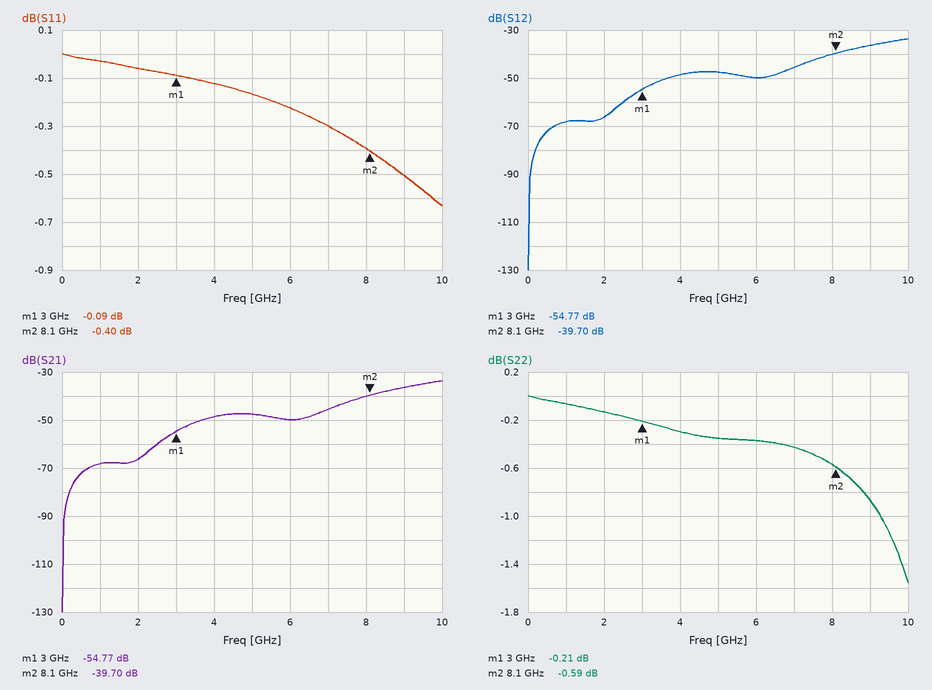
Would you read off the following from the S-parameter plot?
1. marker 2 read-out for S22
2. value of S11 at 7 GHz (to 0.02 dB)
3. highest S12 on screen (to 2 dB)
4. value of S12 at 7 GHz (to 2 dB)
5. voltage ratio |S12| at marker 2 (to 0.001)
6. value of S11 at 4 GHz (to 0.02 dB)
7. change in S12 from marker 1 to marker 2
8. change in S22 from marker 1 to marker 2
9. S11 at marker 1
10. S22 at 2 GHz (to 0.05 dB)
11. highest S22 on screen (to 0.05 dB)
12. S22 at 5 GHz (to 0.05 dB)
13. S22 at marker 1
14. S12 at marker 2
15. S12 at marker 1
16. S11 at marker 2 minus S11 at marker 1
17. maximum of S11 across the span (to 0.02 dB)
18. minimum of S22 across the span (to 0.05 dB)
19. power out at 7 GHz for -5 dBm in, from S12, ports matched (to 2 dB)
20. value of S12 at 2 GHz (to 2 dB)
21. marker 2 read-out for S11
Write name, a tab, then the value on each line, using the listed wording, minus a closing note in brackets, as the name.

marker 2 read-out for S22	-0.59 dB
value of S11 at 7 GHz	-0.30 dB
highest S12 on screen	-34 dB
value of S12 at 7 GHz	-46 dB
voltage ratio |S12| at marker 2	0.010
value of S11 at 4 GHz	-0.12 dB
change in S12 from marker 1 to marker 2	15.07 dB
change in S22 from marker 1 to marker 2	-0.38 dB
S11 at marker 1	-0.09 dB
S22 at 2 GHz	-0.15 dB
highest S22 on screen	0.00 dB
S22 at 5 GHz	-0.35 dB
S22 at marker 1	-0.21 dB
S12 at marker 2	-39.70 dB
S12 at marker 1	-54.77 dB
S11 at marker 2 minus S11 at marker 1	-0.31 dB
maximum of S11 across the span	0.00 dB
minimum of S22 across the span	-1.55 dB
power out at 7 GHz for -5 dBm in, from S12, ports matched	-50 dBm
value of S12 at 2 GHz	-66 dB
marker 2 read-out for S11	-0.40 dB
